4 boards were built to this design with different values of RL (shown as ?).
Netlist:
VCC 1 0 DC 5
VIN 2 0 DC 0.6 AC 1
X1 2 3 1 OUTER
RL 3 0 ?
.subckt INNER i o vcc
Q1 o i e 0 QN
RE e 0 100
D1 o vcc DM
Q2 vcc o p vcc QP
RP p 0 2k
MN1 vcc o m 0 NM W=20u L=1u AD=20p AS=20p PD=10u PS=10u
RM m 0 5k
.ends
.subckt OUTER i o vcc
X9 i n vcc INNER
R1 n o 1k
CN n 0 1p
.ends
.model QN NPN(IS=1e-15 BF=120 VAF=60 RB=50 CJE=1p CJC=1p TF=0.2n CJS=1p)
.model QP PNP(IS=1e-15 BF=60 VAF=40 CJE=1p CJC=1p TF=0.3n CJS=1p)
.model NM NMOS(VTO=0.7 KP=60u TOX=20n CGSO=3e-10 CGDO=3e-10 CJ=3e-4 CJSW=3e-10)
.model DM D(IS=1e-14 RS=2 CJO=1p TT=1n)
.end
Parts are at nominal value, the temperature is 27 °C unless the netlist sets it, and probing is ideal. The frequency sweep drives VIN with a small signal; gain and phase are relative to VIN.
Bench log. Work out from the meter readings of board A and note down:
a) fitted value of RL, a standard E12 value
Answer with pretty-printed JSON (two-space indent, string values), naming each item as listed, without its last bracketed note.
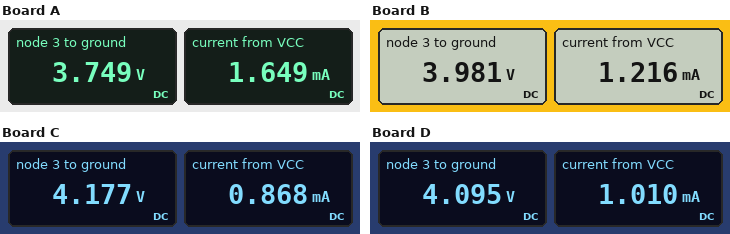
{
  "fitted value of RL, a standard E12 value": "6.8 kΩ"
}
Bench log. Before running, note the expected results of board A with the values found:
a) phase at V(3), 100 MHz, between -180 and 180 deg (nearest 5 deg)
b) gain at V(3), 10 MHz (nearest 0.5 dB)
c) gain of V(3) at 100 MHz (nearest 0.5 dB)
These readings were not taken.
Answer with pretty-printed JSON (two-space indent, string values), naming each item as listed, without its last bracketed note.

{
  "phase at V(3), 100 MHz, between -180 and 180 deg": "110 deg",
  "gain at V(3), 10 MHz": "-35.0 dB",
  "gain of V(3) at 100 MHz": "-36.0 dB"
}
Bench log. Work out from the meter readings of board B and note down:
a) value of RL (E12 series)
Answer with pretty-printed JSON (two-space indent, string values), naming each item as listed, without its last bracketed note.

{
  "value of RL": "12 kΩ"
}
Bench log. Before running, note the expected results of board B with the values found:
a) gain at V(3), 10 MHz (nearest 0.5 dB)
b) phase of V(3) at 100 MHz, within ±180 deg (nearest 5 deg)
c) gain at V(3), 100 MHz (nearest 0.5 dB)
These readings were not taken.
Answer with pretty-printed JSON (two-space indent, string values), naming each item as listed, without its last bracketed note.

{
  "gain at V(3), 10 MHz": "-30.5 dB",
  "phase of V(3) at 100 MHz, within ±180 deg": "105 deg",
  "gain at V(3), 100 MHz": "-31.5 dB"
}
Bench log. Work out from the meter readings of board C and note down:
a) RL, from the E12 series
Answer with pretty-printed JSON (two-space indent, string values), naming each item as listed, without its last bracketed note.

{
  "RL, from the E12 series": "27 kΩ"
}
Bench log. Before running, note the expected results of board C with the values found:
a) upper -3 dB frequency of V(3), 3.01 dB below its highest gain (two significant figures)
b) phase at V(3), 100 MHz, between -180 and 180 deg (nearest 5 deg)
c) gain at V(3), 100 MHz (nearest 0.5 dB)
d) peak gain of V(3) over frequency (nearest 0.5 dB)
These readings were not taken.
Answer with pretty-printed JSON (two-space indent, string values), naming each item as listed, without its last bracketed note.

{
  "upper -3 dB frequency of V(3), 3.01 dB below its highest gain": "6.2 GHz",
  "phase at V(3), 100 MHz, between -180 and 180 deg": "95 deg",
  "gain at V(3), 100 MHz": "-26.0 dB",
  "peak gain of V(3) over frequency": "-23.0 dB"
}
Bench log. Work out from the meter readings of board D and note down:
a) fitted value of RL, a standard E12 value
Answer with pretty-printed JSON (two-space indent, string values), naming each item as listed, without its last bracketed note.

{
  "fitted value of RL, a standard E12 value": "18 kΩ"
}
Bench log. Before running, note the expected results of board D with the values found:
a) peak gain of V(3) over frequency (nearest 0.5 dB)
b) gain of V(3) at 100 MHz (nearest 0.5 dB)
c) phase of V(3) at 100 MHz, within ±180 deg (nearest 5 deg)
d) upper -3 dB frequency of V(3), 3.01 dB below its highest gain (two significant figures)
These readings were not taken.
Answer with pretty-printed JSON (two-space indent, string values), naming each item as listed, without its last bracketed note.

{
  "peak gain of V(3) over frequency": "-24.0 dB",
  "gain of V(3) at 100 MHz": "-28.5 dB",
  "phase of V(3) at 100 MHz, within ±180 deg": "100 deg",
  "upper -3 dB frequency of V(3), 3.01 dB below its highest gain": "8.0 GHz"
}
